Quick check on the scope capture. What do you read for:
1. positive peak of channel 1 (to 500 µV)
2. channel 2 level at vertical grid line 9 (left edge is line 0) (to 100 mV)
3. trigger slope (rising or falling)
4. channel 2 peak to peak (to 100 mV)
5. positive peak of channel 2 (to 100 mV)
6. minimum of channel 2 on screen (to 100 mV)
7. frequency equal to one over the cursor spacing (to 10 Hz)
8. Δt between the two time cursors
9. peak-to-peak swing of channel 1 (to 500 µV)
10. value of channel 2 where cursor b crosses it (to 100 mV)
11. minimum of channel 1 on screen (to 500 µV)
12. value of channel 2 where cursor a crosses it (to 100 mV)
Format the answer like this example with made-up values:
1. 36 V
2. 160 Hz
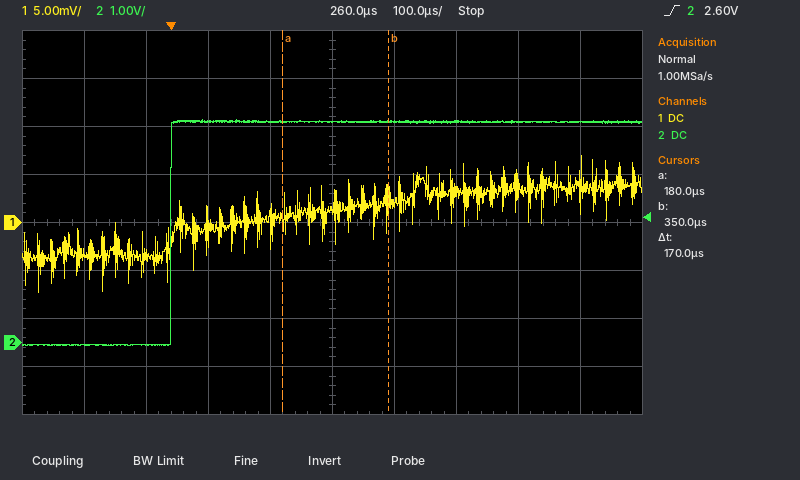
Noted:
1. 7.0 mV
2. 4.6 V
3. rising
4. 4.7 V
5. 4.6 V
6. -100 mV
7. 5.88 kHz
8. 170 µs
9. 14.5 mV
10. 4.6 V
11. -7.5 mV
12. 4.6 V
